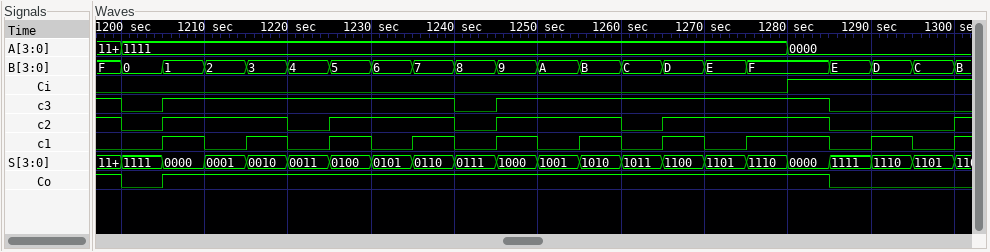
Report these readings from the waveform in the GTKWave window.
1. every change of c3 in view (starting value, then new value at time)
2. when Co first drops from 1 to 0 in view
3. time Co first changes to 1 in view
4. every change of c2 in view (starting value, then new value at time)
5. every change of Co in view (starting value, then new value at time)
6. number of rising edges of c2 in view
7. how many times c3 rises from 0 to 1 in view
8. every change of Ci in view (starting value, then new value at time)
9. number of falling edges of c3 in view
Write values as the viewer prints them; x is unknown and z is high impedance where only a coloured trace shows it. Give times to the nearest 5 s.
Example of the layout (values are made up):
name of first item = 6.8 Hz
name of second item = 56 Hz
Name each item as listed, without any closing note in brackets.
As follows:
every change of c3 in view = 1, 0 at 1200 s, 1 at 1205 s, 0 at 1240 s, 1 at 1245 s, 0 at 1285 s
when Co first drops from 1 to 0 in view = 1200 s
time Co first changes to 1 in view = 1205 s
every change of c2 in view = 1, 0 at 1200 s, 1 at 1205 s, 0 at 1220 s, 1 at 1225 s, 0 at 1240 s, 1 at 1245 s, 0 at 1260 s, 1 at 1265 s, 0 at 1285 s, 1 at 1300 s
every change of Co in view = 1, 0 at 1200 s, 1 at 1205 s, 0 at 1285 s
number of rising edges of c2 in view = 5
how many times c3 rises from 0 to 1 in view = 2
every change of Ci in view = 0, 1 at 1280 s
number of falling edges of c3 in view = 3
